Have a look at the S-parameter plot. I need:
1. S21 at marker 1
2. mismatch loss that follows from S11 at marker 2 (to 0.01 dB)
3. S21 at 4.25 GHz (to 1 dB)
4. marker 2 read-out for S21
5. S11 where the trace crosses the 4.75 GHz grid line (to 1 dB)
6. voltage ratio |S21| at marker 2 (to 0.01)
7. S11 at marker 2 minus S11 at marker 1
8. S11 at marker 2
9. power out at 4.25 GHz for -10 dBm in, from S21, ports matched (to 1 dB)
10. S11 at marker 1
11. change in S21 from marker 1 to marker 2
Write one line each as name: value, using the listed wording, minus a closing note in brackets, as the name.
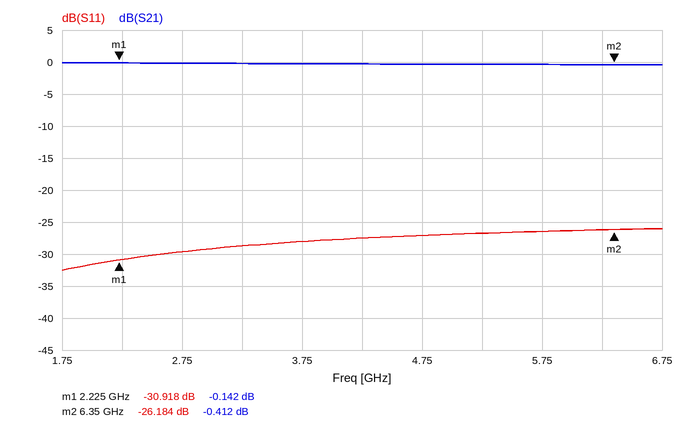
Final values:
S21 at marker 1: -0.142 dB
mismatch loss that follows from S11 at marker 2: 0.01 dB
S21 at 4.25 GHz: 0 dB
marker 2 read-out for S21: -0.412 dB
S11 where the trace crosses the 4.75 GHz grid line: -27 dB
voltage ratio |S21| at marker 2: 0.95
S11 at marker 2 minus S11 at marker 1: 4.734 dB
S11 at marker 2: -26.184 dB
power out at 4.25 GHz for -10 dBm in, from S21, ports matched: -10 dBm
S11 at marker 1: -30.918 dB
change in S21 from marker 1 to marker 2: -0.270 dB
